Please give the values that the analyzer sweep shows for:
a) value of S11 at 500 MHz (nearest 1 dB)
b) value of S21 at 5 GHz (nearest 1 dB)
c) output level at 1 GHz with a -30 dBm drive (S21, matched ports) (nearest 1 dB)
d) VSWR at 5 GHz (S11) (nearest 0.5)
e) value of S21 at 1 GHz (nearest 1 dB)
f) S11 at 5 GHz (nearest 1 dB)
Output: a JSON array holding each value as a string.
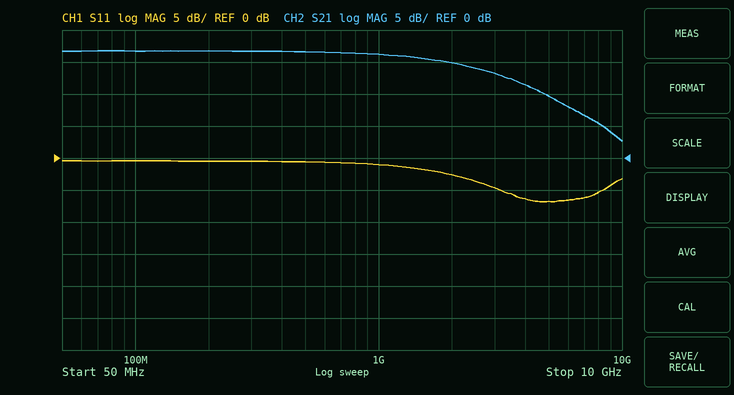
["-1 dB", "10 dB", "-14 dBm", "2.5", "16 dB", "-7 dB"]
